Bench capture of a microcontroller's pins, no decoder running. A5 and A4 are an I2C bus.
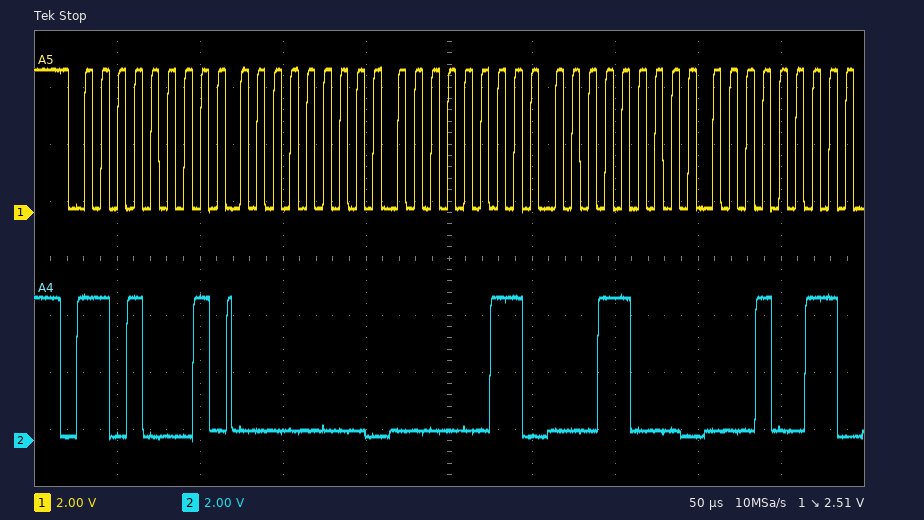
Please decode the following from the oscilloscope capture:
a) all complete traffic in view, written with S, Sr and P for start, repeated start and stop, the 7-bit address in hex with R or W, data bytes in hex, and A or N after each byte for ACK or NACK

S 68R A 00 A 03 A 18 A 13 A
